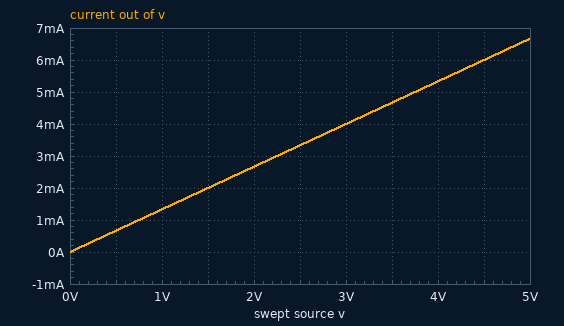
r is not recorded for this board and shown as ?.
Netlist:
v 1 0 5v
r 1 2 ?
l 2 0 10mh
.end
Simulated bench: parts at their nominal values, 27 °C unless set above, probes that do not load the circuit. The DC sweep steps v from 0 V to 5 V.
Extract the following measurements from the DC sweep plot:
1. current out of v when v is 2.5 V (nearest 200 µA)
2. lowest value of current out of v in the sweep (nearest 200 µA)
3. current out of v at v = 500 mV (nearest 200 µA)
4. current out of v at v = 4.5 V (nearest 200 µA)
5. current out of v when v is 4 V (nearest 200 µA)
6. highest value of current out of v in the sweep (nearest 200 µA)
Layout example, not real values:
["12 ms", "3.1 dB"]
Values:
["3.4 mA", "0 A", "600 µA", "6.0 mA", "5.4 mA", "6.6 mA"]
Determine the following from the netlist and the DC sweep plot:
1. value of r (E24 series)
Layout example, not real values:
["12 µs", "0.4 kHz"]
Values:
["750 Ω"]
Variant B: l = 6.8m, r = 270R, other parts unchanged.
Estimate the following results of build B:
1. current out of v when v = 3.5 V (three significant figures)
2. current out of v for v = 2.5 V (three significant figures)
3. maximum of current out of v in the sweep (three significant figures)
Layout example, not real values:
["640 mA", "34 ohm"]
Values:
["13.0 mA", "9.26 mA", "18.5 mA"]
